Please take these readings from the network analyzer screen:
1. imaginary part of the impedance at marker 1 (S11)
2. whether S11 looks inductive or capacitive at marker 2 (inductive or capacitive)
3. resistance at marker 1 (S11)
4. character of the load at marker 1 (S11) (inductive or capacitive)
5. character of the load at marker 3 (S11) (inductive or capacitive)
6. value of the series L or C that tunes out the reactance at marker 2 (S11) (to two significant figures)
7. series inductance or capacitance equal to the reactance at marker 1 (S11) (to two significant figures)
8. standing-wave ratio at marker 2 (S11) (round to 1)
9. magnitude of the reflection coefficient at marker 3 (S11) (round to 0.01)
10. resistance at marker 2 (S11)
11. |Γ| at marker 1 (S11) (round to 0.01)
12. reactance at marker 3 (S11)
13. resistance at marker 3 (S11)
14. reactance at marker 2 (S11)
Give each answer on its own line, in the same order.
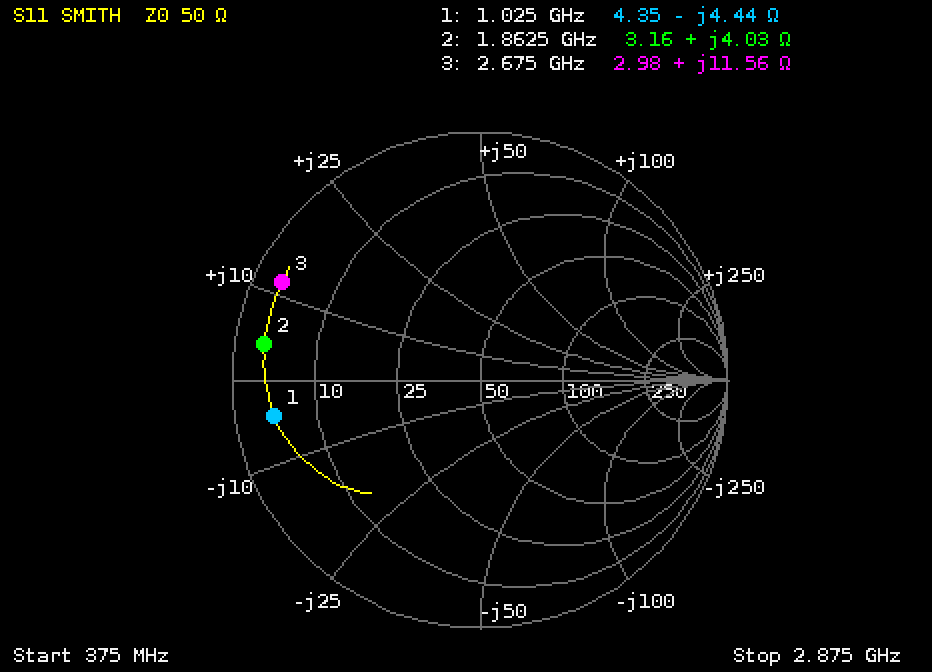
-4.44 Ω
inductive
4.35 Ω
capacitive
inductive
21 pF
35 pF
16
0.89
3.16 Ω
0.84
+11.56 Ω
2.98 Ω
+4.03 Ω
